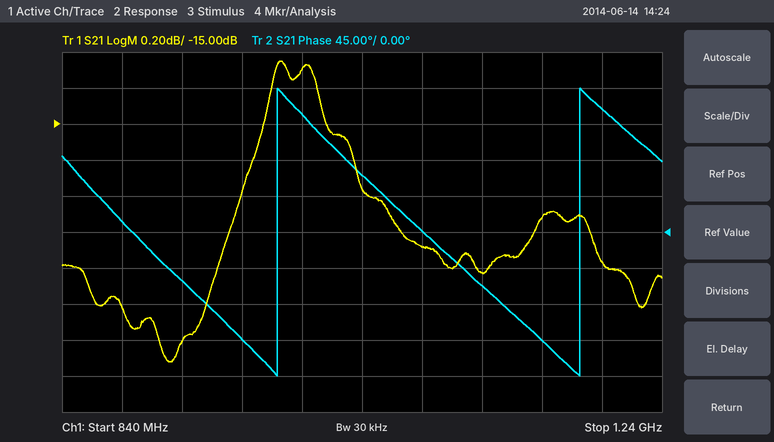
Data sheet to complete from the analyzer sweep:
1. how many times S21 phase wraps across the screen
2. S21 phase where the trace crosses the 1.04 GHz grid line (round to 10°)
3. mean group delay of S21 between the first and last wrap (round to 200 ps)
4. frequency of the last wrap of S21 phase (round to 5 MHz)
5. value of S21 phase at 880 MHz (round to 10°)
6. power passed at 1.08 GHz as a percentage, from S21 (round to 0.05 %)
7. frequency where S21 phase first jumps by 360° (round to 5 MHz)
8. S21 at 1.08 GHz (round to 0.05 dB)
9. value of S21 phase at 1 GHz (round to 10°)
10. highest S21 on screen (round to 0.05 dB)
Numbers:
2
70°
5.0 ns
1.185 GHz
10°
2.70 %
985 MHz
-15.70 dB
150°
-14.65 dB
